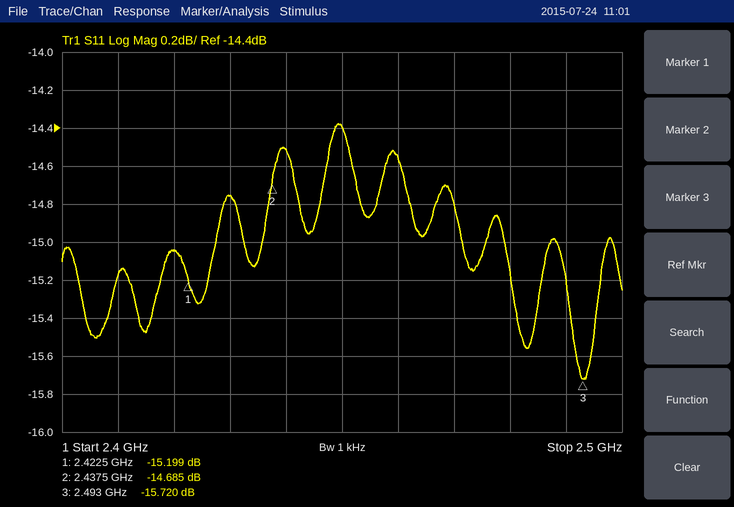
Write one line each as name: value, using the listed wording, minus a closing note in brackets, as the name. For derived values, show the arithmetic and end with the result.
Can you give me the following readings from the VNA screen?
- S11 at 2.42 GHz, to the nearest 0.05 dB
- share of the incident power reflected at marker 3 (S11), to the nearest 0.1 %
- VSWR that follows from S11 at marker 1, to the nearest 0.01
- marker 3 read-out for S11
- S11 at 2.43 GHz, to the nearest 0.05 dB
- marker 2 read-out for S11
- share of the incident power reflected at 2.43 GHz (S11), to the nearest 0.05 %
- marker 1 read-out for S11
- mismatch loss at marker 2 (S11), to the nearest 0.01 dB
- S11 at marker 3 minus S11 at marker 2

S11 at 2.42 GHz, to the nearest 0.05 dB: -15.05 dB
share of the incident power reflected at marker 3 (S11), to the nearest 0.1 %: 10^(-15.72/10) ≈ 2.7 %
VSWR that follows from S11 at marker 1, to the nearest 0.01: (1 + 0.1738)/(1 − 0.1738) ≈ 1.42
marker 3 read-out for S11: -15.720 dB
S11 at 2.43 GHz, to the nearest 0.05 dB: -14.75 dB
marker 2 read-out for S11: -14.685 dB
share of the incident power reflected at 2.43 GHz (S11), to the nearest 0.05 %: 10^(-14.75/10) ≈ 3.35 %
marker 1 read-out for S11: -15.199 dB
mismatch loss at marker 2 (S11), to the nearest 0.01 dB: −10 log10(1 − 10^(-14.685/10)) ≈ 0.15 dB
S11 at marker 3 minus S11 at marker 2: -15.72 − (-14.685) = -1.035 dB
